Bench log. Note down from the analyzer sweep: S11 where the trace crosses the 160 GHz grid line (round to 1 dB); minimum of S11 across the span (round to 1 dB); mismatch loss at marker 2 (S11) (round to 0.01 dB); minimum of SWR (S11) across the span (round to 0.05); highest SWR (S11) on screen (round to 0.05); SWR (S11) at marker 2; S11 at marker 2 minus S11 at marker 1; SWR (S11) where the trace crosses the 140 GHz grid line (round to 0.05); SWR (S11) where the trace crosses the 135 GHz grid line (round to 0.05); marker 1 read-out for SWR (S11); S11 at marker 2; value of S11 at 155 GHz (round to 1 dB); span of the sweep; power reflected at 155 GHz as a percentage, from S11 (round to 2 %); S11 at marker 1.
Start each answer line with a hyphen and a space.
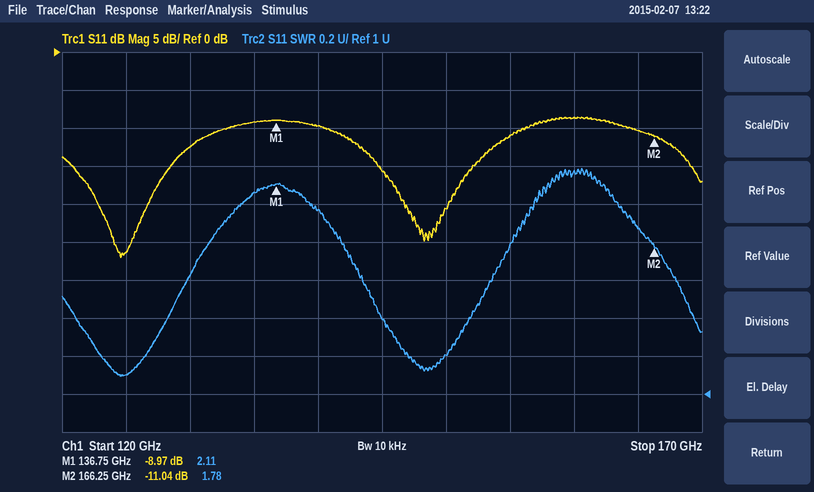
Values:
- -9 dB
- -27 dB
- 0.36 dB
- 1.10
- 2.20
- 1.78
- -2.07 dB
- 1.95
- 2.05
- 2.11
- -11.04 dB
- -11 dB
- 50 GHz
- 8 %
- -8.97 dB
